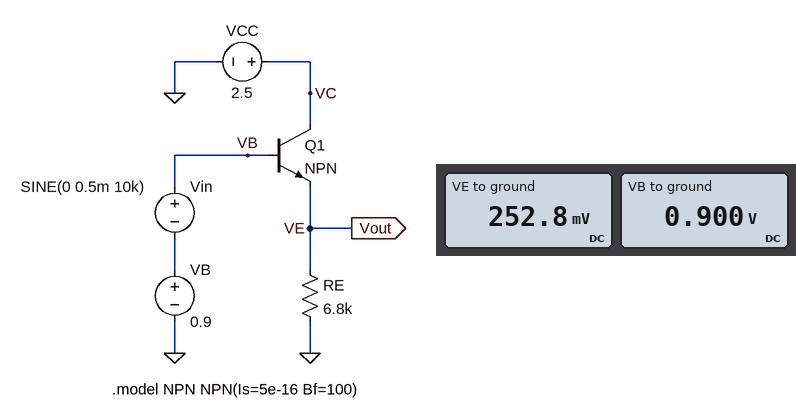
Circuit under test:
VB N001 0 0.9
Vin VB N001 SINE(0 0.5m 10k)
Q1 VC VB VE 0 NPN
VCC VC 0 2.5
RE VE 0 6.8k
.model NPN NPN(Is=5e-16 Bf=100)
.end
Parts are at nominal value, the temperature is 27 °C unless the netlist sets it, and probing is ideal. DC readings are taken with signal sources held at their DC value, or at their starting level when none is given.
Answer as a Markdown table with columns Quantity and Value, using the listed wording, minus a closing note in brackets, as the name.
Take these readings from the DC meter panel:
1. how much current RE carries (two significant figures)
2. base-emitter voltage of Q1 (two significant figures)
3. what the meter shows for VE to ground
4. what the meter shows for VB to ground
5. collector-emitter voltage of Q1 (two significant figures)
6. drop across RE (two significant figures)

| Quantity | Value |
|---|---|
| how much current RE carries | 37 µA |
| base-emitter voltage of Q1 | 650 mV |
| what the meter shows for VE to ground | 252.8 mV |
| what the meter shows for VB to ground | 0.900 V |
| collector-emitter voltage of Q1 | 2.2 V |
| drop across RE | 250 mV |
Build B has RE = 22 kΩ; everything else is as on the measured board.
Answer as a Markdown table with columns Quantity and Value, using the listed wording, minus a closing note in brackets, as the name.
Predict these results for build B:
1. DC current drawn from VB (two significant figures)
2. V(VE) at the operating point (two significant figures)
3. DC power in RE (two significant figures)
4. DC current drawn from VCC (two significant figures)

| Quantity | Value |
|---|---|
| DC current drawn from VB | 130 nA |
| V(VE) at the operating point | 280 mV |
| DC power in RE | 3.6 µW |
| DC current drawn from VCC | 13 µA |
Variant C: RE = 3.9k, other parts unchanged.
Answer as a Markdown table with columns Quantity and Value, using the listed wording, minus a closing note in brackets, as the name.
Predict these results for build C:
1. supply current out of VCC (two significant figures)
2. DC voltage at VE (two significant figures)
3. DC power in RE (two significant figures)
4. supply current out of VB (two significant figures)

| Quantity | Value |
|---|---|
| supply current out of VCC | 61 µA |
| DC voltage at VE | 240 mV |
| DC power in RE | 15 µW |
| supply current out of VB | 610 nA |
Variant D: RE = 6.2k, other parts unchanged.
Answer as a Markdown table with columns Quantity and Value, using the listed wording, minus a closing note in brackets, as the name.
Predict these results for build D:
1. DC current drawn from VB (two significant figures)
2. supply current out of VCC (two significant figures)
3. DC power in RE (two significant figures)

| Quantity | Value |
|---|---|
| DC current drawn from VB | 400 nA |
| supply current out of VCC | 40 µA |
| DC power in RE | 10 µW |
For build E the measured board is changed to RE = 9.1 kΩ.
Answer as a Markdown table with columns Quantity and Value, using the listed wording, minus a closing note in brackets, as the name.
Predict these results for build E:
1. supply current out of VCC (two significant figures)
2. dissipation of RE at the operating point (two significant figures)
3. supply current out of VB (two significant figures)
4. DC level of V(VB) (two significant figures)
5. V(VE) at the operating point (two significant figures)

| Quantity | Value |
|---|---|
| supply current out of VCC | 28 µA |
| dissipation of RE at the operating point | 7.4 µW |
| supply current out of VB | 280 nA |
| DC level of V(VB) | 900 mV |
| V(VE) at the operating point | 260 mV |
